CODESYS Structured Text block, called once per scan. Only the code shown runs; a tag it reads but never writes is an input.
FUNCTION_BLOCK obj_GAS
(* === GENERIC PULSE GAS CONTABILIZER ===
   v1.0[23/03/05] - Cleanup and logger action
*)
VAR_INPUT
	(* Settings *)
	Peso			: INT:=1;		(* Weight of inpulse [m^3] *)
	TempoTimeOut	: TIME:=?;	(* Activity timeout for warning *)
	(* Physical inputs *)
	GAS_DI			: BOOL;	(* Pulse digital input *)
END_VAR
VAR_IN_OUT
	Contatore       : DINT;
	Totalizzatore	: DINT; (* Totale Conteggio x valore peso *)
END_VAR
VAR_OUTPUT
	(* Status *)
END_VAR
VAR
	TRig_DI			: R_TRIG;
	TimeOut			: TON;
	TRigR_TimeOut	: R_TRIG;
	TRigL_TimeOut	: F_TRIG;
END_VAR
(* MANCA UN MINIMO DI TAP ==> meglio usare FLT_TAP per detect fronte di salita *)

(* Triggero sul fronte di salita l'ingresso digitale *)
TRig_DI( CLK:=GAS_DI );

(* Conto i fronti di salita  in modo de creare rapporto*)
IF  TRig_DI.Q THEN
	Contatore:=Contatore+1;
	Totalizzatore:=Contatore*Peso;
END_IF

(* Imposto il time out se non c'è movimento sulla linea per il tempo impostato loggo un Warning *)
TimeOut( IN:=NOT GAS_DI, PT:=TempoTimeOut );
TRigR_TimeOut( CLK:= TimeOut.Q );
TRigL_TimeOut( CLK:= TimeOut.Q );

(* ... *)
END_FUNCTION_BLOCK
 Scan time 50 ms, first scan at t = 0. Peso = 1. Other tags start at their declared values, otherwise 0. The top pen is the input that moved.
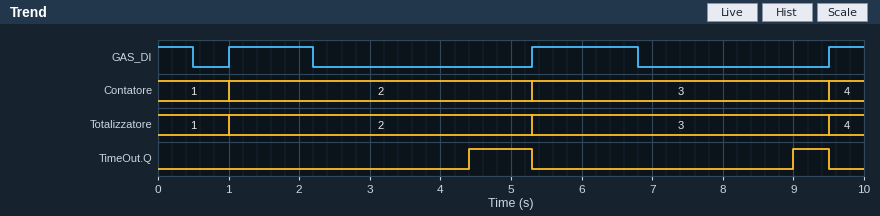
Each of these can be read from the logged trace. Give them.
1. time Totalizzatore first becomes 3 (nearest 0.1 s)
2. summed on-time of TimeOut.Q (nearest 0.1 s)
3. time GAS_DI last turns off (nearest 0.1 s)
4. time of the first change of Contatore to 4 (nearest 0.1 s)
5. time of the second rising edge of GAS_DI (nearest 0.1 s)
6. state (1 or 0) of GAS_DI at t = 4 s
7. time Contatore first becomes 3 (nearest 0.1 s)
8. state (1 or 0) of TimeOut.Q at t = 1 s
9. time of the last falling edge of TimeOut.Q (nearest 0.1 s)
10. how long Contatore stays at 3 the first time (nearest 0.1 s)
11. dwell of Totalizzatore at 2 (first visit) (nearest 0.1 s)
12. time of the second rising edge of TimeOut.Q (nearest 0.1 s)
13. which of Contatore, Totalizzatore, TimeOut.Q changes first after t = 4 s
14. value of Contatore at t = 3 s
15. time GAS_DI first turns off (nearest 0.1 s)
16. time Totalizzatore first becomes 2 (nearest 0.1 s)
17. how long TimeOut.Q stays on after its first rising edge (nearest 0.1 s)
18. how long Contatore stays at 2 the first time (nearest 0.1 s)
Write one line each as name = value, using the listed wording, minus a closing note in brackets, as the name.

time Totalizzatore first becomes 3 = 5.3 s
summed on-time of TimeOut.Q = 1.4 s
time GAS_DI last turns off = 6.8 s
time of the first change of Contatore to 4 = 9.5 s
time of the second rising edge of GAS_DI = 5.3 s
state (1 or 0) of GAS_DI at t = 4 s = 0
time Contatore first becomes 3 = 5.3 s
state (1 or 0) of TimeOut.Q at t = 1 s = 0
time of the last falling edge of TimeOut.Q = 9.5 s
how long Contatore stays at 3 the first time = 4.2 s
dwell of Totalizzatore at 2 (first visit) = 4.3 s
time of the second rising edge of TimeOut.Q = 9.0 s
which of Contatore, Totalizzatore, TimeOut.Q changes first after t = 4 s = TimeOut.Q
value of Contatore at t = 3 s = 2
time GAS_DI first turns off = 0.5 s
time Totalizzatore first becomes 2 = 1.0 s
how long TimeOut.Q stays on after its first rising edge = 0.9 s
how long Contatore stays at 2 the first time = 4.3 s
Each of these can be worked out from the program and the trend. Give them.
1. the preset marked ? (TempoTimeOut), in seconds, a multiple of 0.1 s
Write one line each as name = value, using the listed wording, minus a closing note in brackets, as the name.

the preset marked ? (TempoTimeOut), in seconds, a multiple of 0.1 s = 2.2 s
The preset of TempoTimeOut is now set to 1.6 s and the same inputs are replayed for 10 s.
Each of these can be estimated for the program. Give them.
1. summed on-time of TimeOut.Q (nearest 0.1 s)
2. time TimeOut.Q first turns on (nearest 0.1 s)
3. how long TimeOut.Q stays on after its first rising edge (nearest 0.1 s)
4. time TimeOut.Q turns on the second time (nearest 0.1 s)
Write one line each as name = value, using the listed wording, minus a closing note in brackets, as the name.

summed on-time of TimeOut.Q = 2.6 s
time TimeOut.Q first turns on = 3.8 s
how long TimeOut.Q stays on after its first rising edge = 1.5 s
time TimeOut.Q turns on the second time = 8.4 s
